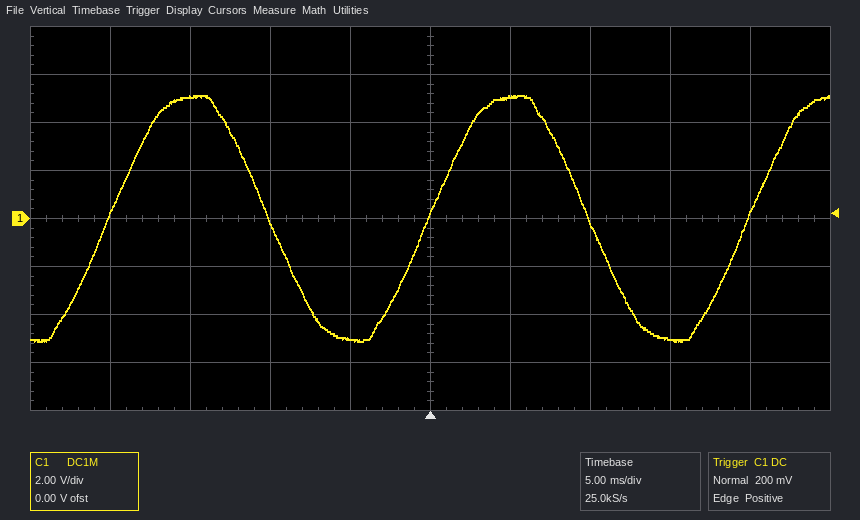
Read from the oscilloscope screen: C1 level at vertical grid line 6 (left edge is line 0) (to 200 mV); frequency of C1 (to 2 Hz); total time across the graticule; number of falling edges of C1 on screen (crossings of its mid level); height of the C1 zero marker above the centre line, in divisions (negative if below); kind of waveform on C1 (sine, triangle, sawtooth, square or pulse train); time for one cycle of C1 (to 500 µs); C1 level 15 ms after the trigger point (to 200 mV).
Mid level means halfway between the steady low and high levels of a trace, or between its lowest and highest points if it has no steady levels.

5.0 V
50 Hz
50 ms
2
0.0 div
sine
20.0 ms
-5.0 V
